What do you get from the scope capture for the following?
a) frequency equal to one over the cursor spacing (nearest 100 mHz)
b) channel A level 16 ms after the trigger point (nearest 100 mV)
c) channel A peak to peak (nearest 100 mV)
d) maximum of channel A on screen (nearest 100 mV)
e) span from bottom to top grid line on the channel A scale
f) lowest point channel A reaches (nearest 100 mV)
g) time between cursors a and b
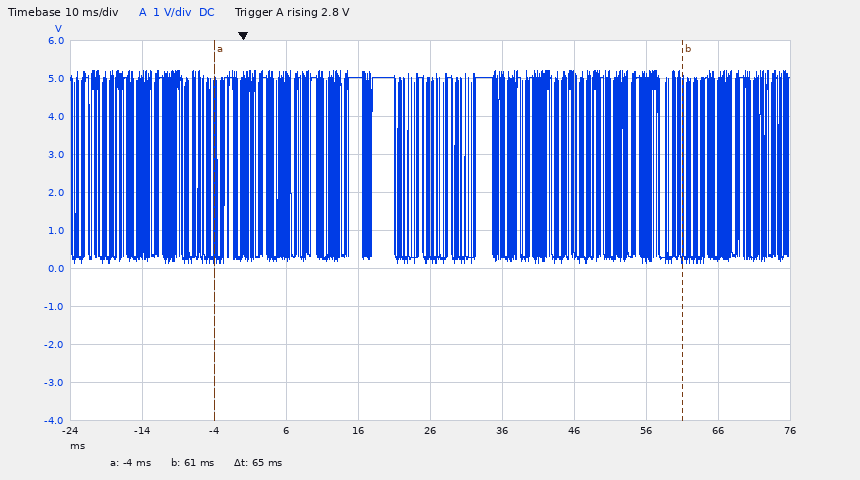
15.4 Hz
5.0 V
5.1 V
5.2 V
10 V
100 mV
65 ms
